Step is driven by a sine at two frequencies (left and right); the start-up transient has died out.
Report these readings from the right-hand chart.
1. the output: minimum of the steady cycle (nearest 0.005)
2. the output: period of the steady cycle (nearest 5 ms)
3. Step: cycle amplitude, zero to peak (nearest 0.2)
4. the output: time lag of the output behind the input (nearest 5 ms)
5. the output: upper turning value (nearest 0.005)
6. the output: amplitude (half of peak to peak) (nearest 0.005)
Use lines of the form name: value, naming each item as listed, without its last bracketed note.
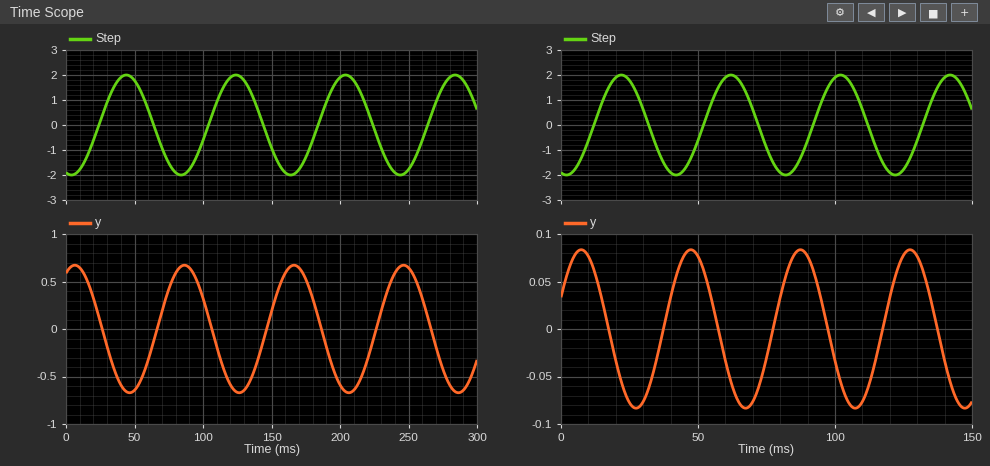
the output: minimum of the steady cycle: -0.085
the output: period of the steady cycle: 40 ms
Step: cycle amplitude, zero to peak: 2.0
the output: time lag of the output behind the input: 25 ms
the output: upper turning value: 0.085
the output: amplitude (half of peak to peak): 0.085
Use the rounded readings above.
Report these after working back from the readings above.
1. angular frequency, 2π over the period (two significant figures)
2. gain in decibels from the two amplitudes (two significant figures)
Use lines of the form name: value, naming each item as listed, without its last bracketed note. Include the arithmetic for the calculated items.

angular frequency, 2π over the period: 2π / 40 = 0.16 rad/ms
gain in decibels from the two amplitudes: 20 log10(0.085 / 2) = -27 dB
